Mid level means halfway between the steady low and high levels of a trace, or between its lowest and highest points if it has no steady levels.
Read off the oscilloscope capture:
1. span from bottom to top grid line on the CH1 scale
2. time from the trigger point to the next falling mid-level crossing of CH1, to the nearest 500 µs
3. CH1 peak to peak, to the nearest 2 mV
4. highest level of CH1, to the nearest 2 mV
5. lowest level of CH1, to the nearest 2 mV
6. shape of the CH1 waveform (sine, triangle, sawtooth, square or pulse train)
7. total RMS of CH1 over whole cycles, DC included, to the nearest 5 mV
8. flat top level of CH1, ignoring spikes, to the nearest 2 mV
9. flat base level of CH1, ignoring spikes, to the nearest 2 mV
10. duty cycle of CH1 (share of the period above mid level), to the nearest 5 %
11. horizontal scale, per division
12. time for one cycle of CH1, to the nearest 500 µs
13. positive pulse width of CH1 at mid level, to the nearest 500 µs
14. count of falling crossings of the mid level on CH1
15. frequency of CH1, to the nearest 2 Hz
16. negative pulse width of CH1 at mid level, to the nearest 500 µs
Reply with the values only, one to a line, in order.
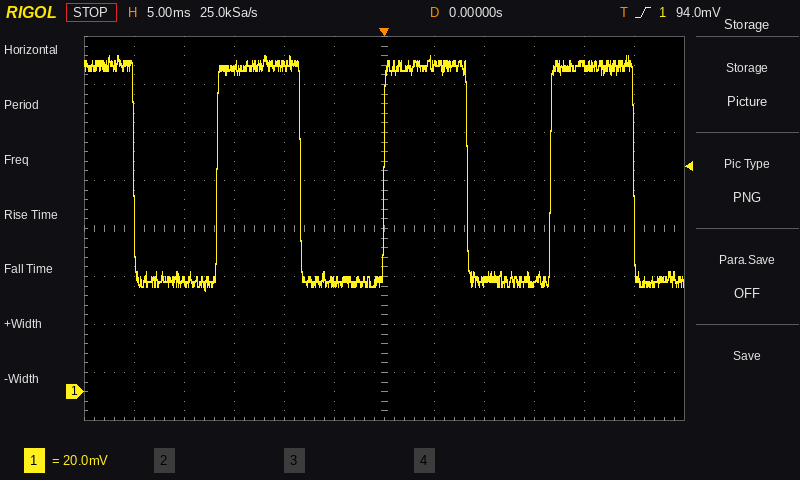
160 mV
8.5 ms
98 mV
140 mV
42 mV
square
100 mV
136 mV
46 mV
50 %
5 ms
16.5 ms
8.5 ms
4
60 Hz
8.5 ms
